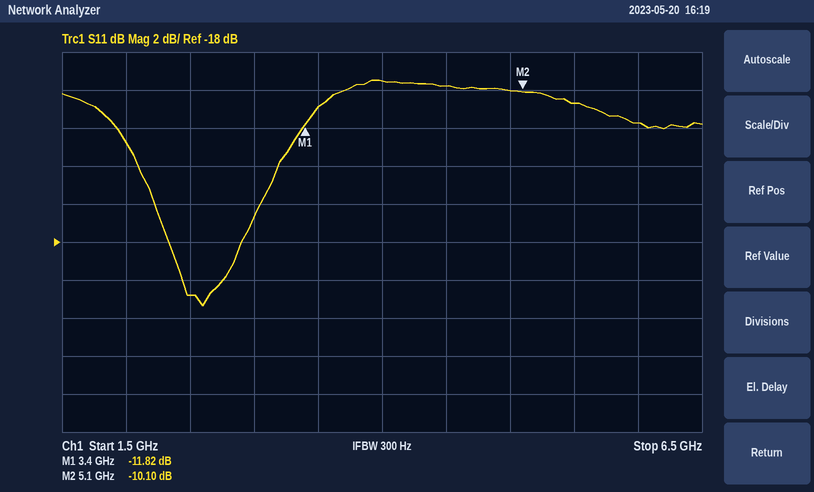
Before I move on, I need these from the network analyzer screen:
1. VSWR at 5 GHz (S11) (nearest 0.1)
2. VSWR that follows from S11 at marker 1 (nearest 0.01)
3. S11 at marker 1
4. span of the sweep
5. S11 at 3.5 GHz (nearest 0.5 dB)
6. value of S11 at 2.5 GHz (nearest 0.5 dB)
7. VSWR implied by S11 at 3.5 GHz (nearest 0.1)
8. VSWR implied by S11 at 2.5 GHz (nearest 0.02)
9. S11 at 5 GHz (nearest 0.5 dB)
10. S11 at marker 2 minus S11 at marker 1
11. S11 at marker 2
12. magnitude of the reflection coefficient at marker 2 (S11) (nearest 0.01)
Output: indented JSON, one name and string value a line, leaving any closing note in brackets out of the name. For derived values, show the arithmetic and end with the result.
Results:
{
  "VSWR at 5 GHz (S11)": "|Γ| = 10^(-10/20) = 0.3162; VSWR = (1 + 0.3162)/(1 − 0.3162) ≈ 1.9",
  "VSWR that follows from S11 at marker 1": "(1 + 0.2564)/(1 − 0.2564) ≈ 1.69",
  "S11 at marker 1": "-11.82 dB",
  "span of the sweep": "5 GHz",
  "S11 at 3.5 GHz": "-11.0 dB",
  "value of S11 at 2.5 GHz": "-21.0 dB",
  "VSWR implied by S11 at 3.5 GHz": "|Γ| = 10^(-11/20) = 0.2818; VSWR = (1 + 0.2818)/(1 − 0.2818) ≈ 1.8",
  "VSWR implied by S11 at 2.5 GHz": "|Γ| = 10^(-21/20) = 0.0891; VSWR = (1 + 0.0891)/(1 − 0.0891) ≈ 1.20",
  "S11 at 5 GHz": "-10.0 dB",
  "S11 at marker 2 minus S11 at marker 1": "-10.1 − (-11.82) = 1.72 dB",
  "S11 at marker 2": "-10.10 dB",
  "magnitude of the reflection coefficient at marker 2 (S11)": "10^(-10.1/20) ≈ 0.31"
}
